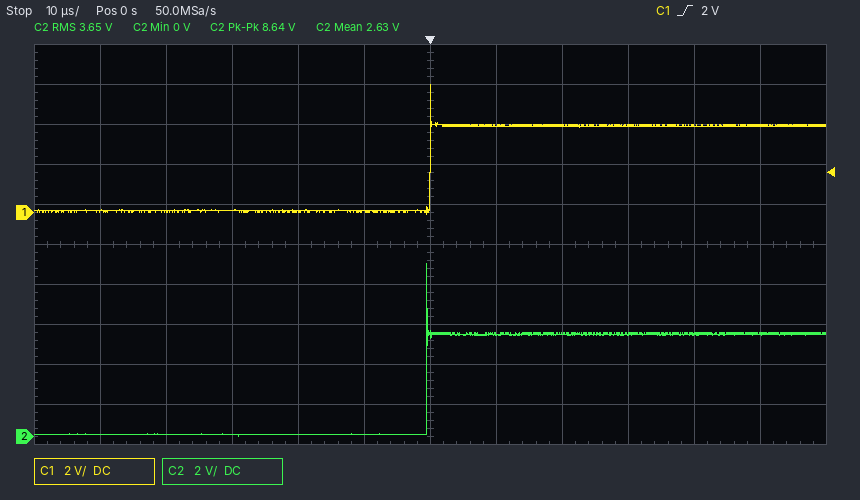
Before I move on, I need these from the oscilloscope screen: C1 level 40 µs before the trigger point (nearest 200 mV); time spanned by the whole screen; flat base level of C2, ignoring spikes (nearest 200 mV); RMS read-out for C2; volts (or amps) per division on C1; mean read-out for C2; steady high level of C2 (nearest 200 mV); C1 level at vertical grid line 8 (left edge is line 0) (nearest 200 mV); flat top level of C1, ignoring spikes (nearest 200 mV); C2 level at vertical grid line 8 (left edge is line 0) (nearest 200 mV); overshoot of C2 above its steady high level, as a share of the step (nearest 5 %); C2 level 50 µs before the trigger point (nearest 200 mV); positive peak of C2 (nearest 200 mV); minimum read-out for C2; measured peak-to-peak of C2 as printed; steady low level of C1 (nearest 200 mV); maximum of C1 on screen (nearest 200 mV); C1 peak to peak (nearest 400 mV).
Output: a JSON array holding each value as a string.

["0.0 V", "120 µs", "0.0 V", "3.65 V", "2 V", "2.63 V", "5.2 V", "4.4 V", "4.4 V", "5.2 V", "70 %", "0.0 V", "8.6 V", "0 V", "8.64 V", "0.0 V", "6.4 V", "6.4 V"]
